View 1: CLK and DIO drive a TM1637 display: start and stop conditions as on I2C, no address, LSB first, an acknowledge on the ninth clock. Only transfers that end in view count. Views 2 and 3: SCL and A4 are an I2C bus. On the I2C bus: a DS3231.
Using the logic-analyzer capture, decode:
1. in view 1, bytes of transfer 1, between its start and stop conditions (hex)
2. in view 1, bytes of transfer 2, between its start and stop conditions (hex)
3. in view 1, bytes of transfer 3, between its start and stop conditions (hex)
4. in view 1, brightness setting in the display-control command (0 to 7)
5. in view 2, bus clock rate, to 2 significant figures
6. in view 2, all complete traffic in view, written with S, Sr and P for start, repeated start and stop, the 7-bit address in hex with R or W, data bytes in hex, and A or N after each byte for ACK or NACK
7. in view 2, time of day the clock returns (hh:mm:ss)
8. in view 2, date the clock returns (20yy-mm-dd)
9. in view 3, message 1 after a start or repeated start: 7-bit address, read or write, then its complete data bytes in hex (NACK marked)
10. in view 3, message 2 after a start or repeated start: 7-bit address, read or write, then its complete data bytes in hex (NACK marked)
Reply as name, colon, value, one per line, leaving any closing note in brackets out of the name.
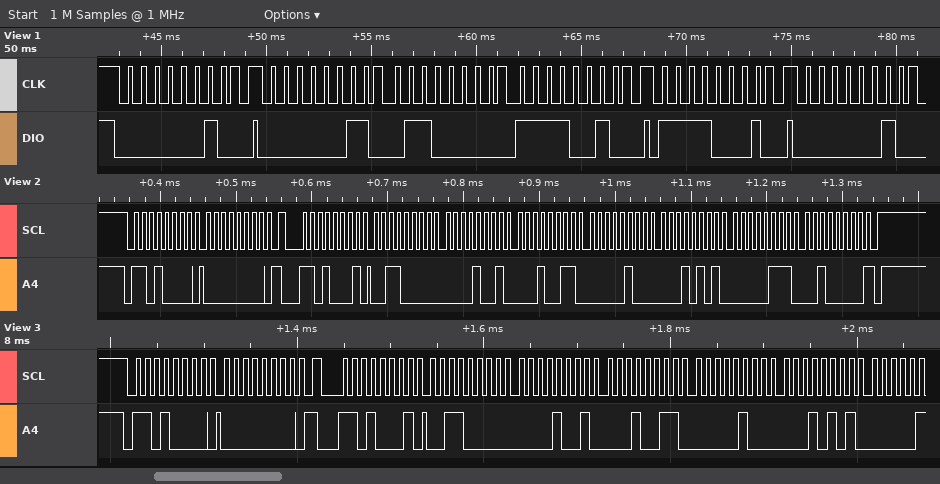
in view 1, bytes of transfer 1, between its start and stop conditions: 40
in view 1, bytes of transfer 2, between its start and stop conditions: C0 06 4F
in view 1, bytes of transfer 3, between its start and stop conditions: 8F
in view 1, brightness setting in the display-control command: 7
in view 2, bus clock rate, to 2 significant figures: 100 kHz
in view 2, all complete traffic in view, written with S, Sr and P for start, repeated start and stop, the 7-bit address in hex with R or W, data bytes in hex, and A or N after each byte for ACK or NACK: S 68W A 00 A Sr 68R A 30 A 09 A 13 A 04 A 15 A 07 A 20 N P
in view 2, time of day the clock returns: 13:09:30
in view 2, date the clock returns: 2020-07-15
in view 3, message 1 after a start or repeated start: 7-bit address, read or write, then its complete data bytes in hex: 0x68 write: 00
in view 3, message 2 after a start or repeated start: 7-bit address, read or write, then its complete data bytes in hex: 0x68 read: 30 09 13 04 15
